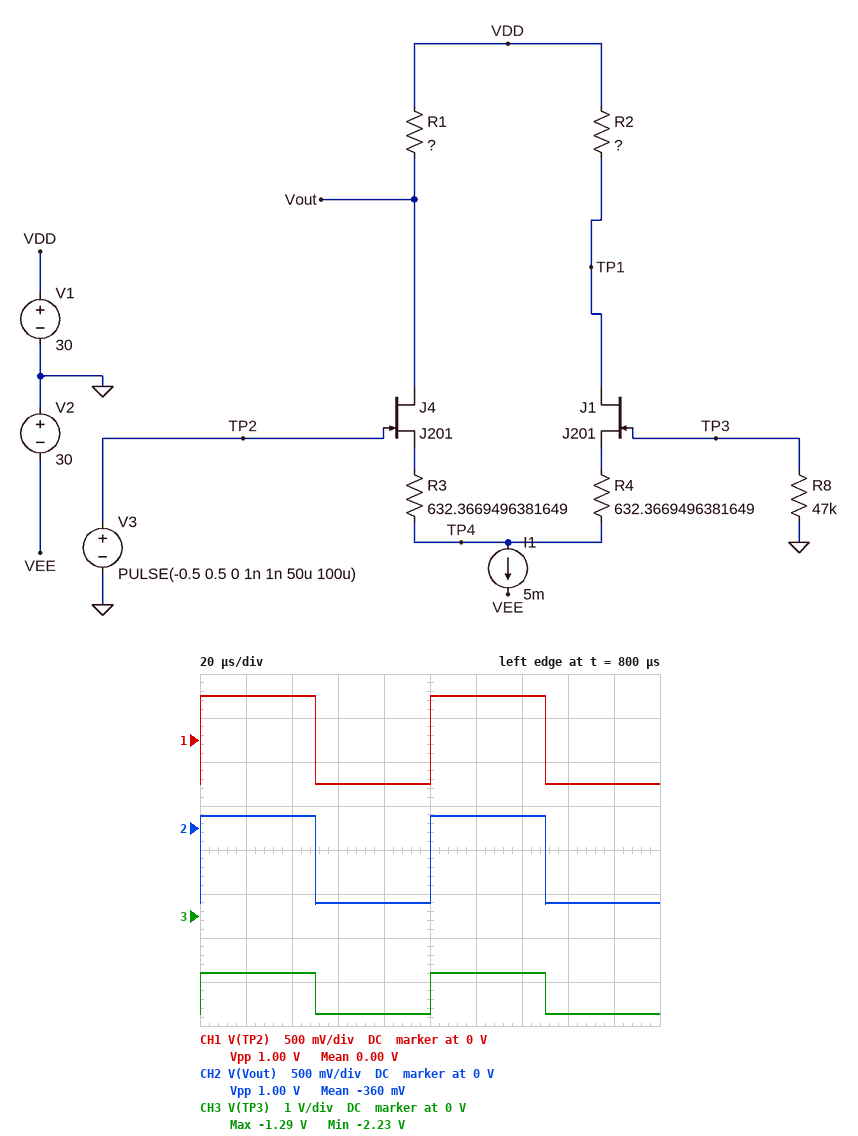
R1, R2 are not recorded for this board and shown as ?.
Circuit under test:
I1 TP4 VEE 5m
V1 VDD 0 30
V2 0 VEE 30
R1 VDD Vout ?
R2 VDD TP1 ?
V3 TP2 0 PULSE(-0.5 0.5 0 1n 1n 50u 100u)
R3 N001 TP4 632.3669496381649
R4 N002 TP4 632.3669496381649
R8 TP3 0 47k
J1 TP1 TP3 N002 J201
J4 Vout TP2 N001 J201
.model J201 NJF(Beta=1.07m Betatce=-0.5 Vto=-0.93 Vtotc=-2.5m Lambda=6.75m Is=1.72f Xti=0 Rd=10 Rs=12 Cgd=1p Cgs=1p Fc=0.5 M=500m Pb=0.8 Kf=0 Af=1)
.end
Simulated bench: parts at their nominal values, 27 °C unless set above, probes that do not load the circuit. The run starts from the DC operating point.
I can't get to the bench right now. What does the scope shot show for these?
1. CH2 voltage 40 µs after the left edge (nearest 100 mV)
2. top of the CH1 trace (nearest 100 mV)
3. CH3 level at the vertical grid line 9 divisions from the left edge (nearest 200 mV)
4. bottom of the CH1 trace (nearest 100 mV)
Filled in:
100 mV
500 mV
-2.2 V
-500 mV
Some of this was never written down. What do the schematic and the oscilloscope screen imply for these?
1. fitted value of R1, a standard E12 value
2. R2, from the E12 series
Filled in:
27 kΩ
27 kΩ
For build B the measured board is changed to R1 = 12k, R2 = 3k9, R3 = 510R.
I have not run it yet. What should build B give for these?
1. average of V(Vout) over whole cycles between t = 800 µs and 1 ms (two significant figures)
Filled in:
1.1 V
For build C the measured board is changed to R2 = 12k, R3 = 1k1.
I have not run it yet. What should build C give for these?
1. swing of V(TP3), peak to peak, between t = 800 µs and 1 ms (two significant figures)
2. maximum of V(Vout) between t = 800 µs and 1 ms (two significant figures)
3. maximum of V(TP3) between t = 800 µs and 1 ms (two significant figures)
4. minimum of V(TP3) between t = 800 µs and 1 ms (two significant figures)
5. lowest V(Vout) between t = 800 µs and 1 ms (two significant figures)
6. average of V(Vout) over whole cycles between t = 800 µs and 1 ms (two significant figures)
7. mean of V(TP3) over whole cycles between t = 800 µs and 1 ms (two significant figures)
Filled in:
840 mV
160 mV
-760 mV
-1.6 V
-840 mV
-340 mV
-1.2 V
